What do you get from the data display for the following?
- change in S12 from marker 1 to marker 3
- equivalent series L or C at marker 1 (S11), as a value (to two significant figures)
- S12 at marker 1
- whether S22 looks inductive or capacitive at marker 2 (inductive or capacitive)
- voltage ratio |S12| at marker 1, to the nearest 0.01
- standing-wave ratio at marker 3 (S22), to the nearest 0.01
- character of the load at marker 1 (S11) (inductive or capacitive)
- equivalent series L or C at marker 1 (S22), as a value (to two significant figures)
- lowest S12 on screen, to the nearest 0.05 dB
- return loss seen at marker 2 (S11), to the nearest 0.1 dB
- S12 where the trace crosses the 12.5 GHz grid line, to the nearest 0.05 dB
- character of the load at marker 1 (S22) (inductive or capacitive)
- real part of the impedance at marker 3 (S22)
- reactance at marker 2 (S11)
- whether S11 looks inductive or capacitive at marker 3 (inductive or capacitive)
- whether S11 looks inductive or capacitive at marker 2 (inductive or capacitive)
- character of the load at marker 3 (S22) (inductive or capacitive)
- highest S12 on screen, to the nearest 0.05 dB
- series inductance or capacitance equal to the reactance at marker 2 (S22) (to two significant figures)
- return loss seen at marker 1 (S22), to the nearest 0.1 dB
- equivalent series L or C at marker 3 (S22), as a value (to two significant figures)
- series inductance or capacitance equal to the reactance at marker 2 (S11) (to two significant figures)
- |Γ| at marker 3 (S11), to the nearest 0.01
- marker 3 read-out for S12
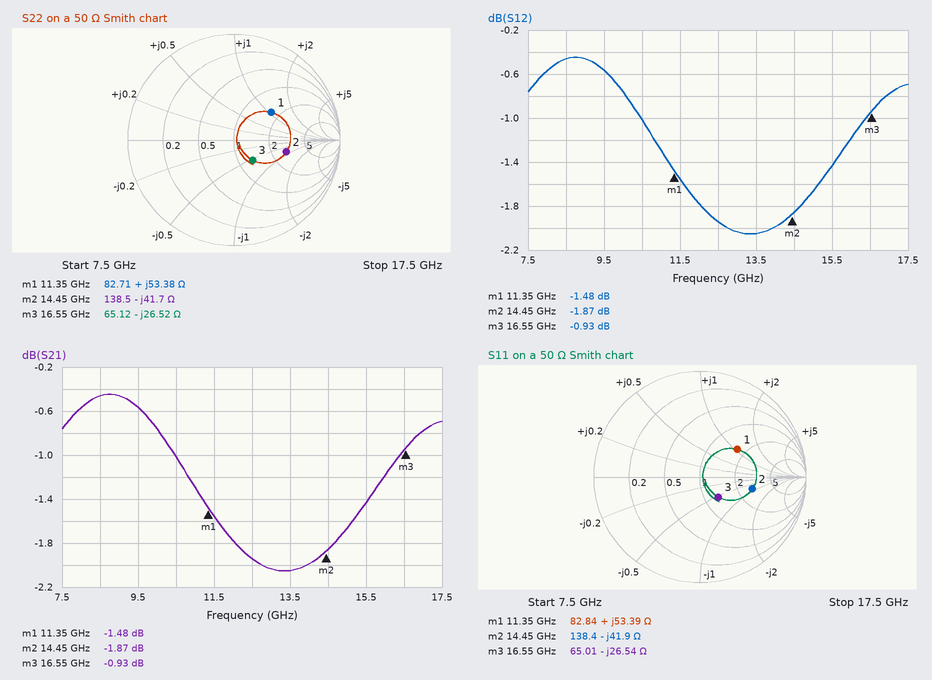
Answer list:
0.55 dB
750 pH
-1.48 dB
capacitive
0.84
1.70
inductive
750 pH
-2.05 dB
5.9 dB
-1.95 dB
inductive
65.12 Ω
-41.9 Ω
capacitive
capacitive
capacitive
-0.45 dB
260 fF
7.2 dB
360 fF
260 fF
0.26
-0.93 dB
